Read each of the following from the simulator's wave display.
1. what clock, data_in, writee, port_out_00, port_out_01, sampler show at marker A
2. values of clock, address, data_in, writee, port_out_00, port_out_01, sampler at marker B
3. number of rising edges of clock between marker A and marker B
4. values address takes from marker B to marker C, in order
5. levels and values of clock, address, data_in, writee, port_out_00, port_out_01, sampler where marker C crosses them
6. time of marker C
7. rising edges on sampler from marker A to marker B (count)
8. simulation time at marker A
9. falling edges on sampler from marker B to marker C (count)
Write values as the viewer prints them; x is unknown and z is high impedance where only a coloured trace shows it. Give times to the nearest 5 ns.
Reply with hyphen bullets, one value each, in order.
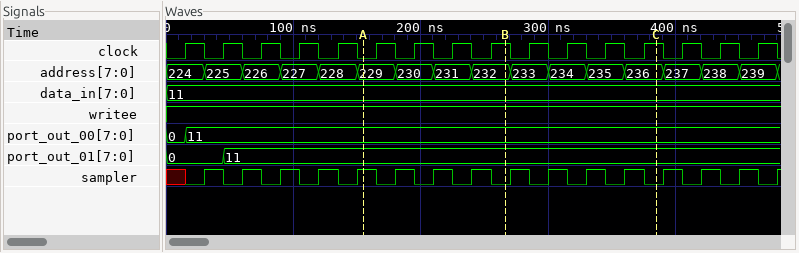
- clock=0, data_in=11, writee=1, port_out_00=11, port_out_01=11, sampler=1
- clock=1, address=232, data_in=11, writee=1, port_out_00=11, port_out_01=11, sampler=0
- 4
- 232, 233, 234, 235, 236
- clock=1, address=236, data_in=11, writee=1, port_out_00=11, port_out_01=11, sampler=0
- 385 ns
- 3
- 155 ns
- 4
